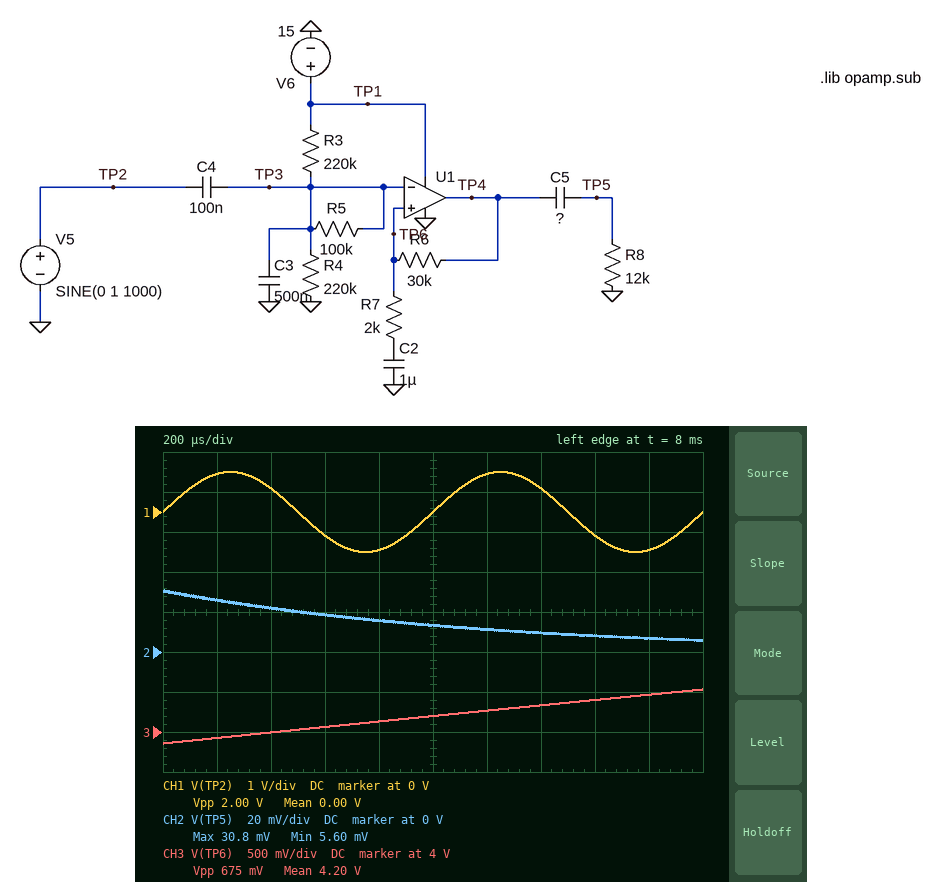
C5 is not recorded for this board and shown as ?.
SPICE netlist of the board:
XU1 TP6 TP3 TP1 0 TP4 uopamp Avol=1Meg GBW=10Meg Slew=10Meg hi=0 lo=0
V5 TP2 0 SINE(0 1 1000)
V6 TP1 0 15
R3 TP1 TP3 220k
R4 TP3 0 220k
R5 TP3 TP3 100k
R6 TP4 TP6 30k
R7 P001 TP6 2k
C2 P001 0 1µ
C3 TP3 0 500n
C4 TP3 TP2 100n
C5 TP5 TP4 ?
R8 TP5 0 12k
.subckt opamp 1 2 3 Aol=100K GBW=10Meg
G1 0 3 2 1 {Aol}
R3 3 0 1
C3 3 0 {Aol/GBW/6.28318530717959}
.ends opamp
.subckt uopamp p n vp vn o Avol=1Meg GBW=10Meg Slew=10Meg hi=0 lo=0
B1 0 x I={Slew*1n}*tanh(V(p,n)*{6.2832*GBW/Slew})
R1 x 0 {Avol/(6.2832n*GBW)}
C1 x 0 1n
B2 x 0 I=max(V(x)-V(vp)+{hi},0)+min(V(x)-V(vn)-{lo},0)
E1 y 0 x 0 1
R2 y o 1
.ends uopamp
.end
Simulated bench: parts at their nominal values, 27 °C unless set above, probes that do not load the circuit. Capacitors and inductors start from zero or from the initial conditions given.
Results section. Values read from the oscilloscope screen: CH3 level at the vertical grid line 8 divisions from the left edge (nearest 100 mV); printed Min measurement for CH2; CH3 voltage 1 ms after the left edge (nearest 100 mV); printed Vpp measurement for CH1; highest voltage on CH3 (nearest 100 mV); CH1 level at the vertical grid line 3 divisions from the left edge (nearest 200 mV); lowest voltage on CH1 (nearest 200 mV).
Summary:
4.4 V
5.60 mV
4.2 V
2.00 V
4.5 V
-600 mV
-1.0 V
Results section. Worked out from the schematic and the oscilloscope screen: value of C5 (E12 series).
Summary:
100 nF
